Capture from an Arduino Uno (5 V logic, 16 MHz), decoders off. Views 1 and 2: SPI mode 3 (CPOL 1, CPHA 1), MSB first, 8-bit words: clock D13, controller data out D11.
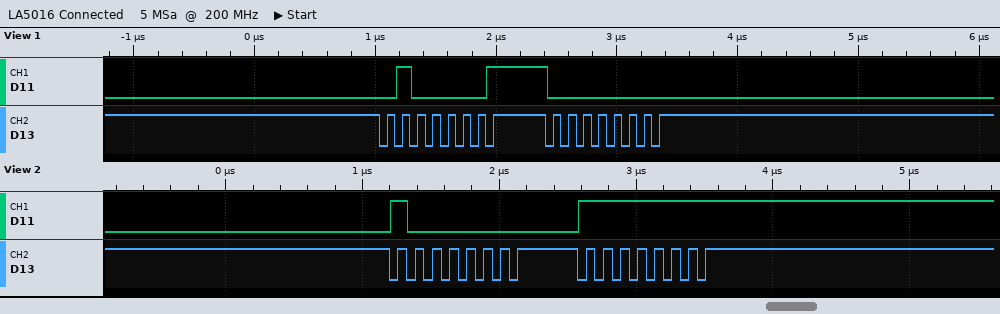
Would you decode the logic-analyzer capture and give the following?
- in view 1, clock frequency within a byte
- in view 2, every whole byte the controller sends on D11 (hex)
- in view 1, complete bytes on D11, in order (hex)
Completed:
8 MHz
80 FF
41 00
